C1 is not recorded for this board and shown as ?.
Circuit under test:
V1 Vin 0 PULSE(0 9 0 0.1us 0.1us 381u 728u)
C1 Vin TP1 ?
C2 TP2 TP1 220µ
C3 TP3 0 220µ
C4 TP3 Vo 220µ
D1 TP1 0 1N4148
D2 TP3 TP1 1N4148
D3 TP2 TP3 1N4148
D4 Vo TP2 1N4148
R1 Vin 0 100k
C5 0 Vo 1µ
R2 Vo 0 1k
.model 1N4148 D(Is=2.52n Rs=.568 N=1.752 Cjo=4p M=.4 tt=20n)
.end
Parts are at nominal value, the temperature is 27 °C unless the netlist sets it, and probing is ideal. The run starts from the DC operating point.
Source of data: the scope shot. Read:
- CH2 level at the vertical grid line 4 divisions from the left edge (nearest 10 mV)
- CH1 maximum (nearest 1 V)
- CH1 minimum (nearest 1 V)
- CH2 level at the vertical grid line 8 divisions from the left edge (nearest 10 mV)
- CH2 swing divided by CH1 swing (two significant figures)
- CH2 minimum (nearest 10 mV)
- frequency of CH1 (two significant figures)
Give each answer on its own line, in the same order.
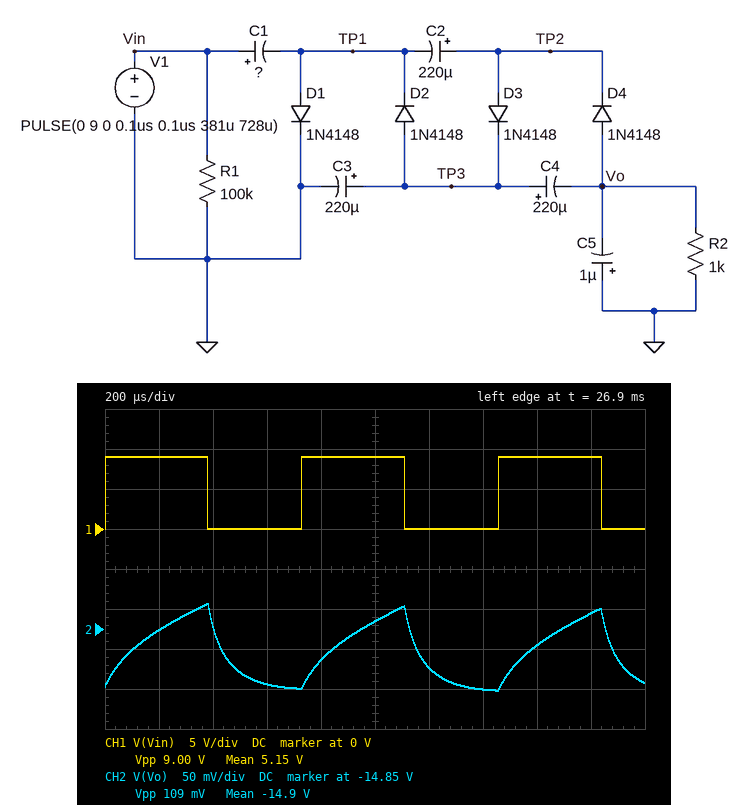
-14.89 V
9 V
0 V
-14.87 V
0.012
-14.93 V
1.4 kHz
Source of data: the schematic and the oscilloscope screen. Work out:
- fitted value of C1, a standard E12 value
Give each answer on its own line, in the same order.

330 µF
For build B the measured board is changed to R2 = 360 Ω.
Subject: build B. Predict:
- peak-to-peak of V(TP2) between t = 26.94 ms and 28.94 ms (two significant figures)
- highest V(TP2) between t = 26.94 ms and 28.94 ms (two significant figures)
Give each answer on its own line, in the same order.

9.3 V
-6.1 V
